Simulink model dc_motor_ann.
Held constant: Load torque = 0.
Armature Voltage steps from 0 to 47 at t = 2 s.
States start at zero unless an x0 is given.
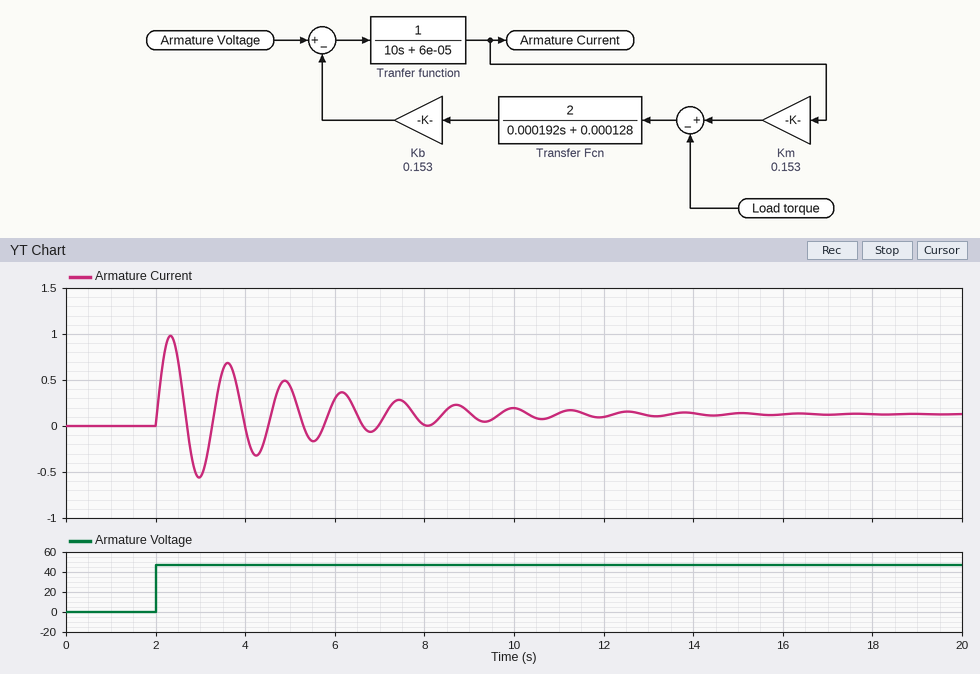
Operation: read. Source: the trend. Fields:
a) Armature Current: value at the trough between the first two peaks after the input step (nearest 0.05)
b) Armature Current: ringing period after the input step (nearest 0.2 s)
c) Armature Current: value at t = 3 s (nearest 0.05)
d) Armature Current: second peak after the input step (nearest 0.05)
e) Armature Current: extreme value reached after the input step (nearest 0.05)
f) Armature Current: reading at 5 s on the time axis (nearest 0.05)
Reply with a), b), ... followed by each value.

a) -0.55
b) 1.2 s
c) -0.55
d) 0.70
e) 1.00
f) 0.45
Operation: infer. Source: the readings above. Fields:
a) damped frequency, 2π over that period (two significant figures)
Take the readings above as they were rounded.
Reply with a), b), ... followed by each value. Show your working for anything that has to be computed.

a) 2π / 1.2 = 5.2 rad/s
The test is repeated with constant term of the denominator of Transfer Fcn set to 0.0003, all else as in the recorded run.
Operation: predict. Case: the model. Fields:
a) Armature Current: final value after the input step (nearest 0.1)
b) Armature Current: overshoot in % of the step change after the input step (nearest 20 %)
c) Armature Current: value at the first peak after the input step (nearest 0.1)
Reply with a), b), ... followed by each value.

a) 0.3
b) 240 %
c) 1.0
